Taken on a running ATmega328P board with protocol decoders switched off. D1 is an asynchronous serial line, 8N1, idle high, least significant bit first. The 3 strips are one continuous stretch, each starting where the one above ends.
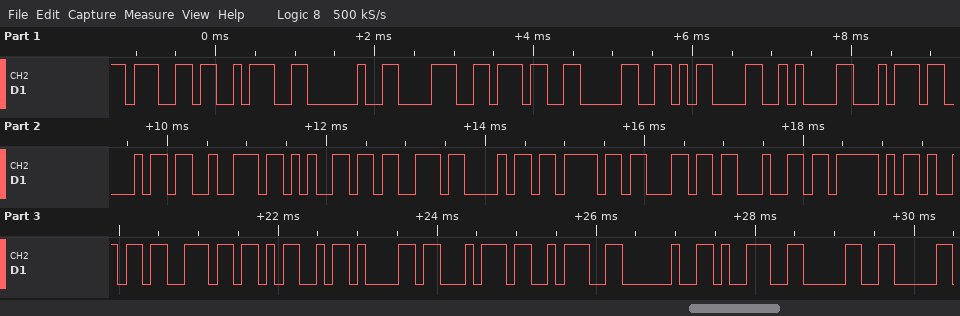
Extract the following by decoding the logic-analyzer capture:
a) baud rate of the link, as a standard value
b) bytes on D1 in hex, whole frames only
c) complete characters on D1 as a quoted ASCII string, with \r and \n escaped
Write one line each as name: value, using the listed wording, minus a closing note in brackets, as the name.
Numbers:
baud rate of the link, as a standard value: 9600 baud
bytes on D1 in hex, whole frames only: 0x67 0x3A 0x20 0x38 0x37 0x30 0x0D 0x0A 0x74 0x68 0x72 0x65 0x73 0x68 0x6F 0x6C 0x64 0x5F 0x69 0x6E 0x4D 0x61 0x74 0x3A 0x20 0x39 0x30
complete characters on D1 as a quoted ASCII string, with \r and \n escaped: "g: 870\r\nthreshold_inMat: 90"
